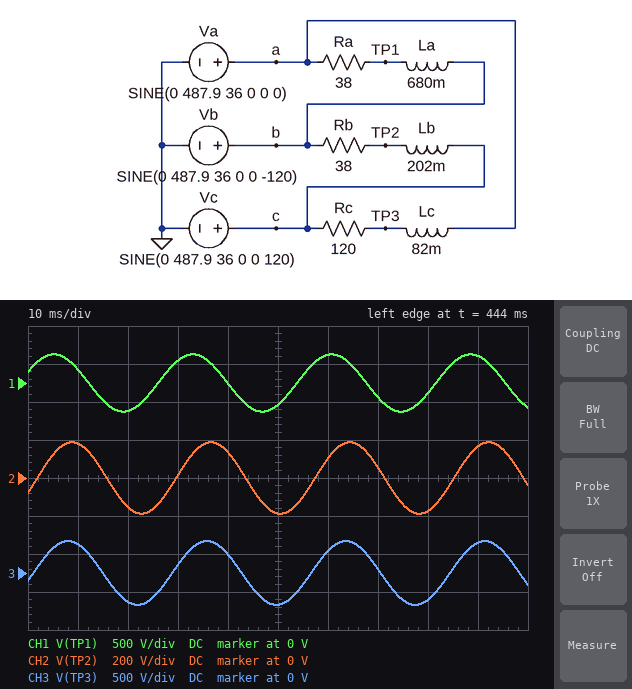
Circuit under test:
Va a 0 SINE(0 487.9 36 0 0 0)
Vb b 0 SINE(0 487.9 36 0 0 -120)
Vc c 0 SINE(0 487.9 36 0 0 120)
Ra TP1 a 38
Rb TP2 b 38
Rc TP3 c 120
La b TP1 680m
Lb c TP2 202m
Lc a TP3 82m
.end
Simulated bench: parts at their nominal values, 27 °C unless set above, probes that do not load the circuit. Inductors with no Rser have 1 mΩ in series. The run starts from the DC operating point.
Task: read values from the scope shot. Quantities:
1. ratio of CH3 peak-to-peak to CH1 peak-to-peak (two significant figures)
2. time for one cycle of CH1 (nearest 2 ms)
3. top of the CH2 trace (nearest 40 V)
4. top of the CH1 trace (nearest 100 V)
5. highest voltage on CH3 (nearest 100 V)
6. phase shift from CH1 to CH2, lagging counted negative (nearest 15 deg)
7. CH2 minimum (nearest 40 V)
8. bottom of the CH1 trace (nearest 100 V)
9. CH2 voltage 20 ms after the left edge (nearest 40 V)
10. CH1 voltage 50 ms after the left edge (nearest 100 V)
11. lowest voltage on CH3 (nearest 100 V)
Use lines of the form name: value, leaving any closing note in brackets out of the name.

ratio of CH3 peak-to-peak to CH1 peak-to-peak: 1.1
time for one cycle of CH1: 28 ms
top of the CH2 trace: 200 V
top of the CH1 trace: 400 V
highest voltage on CH3: 400 V
phase shift from CH1 to CH2, lagging counted negative: -45 deg
CH2 minimum: -200 V
bottom of the CH1 trace: -400 V
CH2 voltage 20 ms after the left edge: -160 V
CH1 voltage 50 ms after the left edge: -300 V
lowest voltage on CH3: -400 V
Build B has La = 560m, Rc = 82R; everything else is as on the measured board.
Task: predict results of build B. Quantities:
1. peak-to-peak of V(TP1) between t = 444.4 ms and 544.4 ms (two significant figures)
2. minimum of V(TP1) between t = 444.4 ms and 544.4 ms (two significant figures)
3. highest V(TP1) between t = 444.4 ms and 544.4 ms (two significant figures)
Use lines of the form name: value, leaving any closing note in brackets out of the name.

peak-to-peak of V(TP1) between t = 444.4 ms and 544.4 ms: 710 V
minimum of V(TP1) between t = 444.4 ms and 544.4 ms: -350 V
highest V(TP1) between t = 444.4 ms and 544.4 ms: 350 V
